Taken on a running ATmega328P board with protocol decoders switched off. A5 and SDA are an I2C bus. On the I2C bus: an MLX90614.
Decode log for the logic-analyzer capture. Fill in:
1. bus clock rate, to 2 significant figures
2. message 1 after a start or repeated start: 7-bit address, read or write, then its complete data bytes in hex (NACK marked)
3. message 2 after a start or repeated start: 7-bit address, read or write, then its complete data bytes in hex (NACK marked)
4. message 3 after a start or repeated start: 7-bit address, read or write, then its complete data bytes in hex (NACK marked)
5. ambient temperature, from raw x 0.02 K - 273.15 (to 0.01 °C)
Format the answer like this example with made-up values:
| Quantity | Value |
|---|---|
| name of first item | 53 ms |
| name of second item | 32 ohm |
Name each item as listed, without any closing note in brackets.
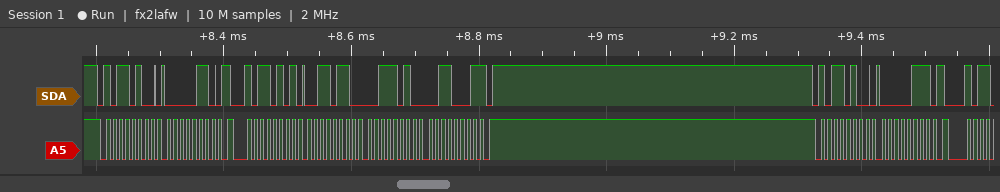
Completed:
| Quantity | Value |
|---|---|
| bus clock rate, to 2 significant figures | 100 kHz |
| message 1 after a start or repeated start: 7-bit address, read or write, then its complete data bytes in hex | 0x5A write: 06 |
| message 2 after a start or repeated start: 7-bit address, read or write, then its complete data bytes in hex | 0x5A read: 36 3A 31 NACK |
| message 3 after a start or repeated start: 7-bit address, read or write, then its complete data bytes in hex | 0x5A write: 07 |
| ambient temperature, from raw x 0.02 K - 273.15 | 24.89 °C |
